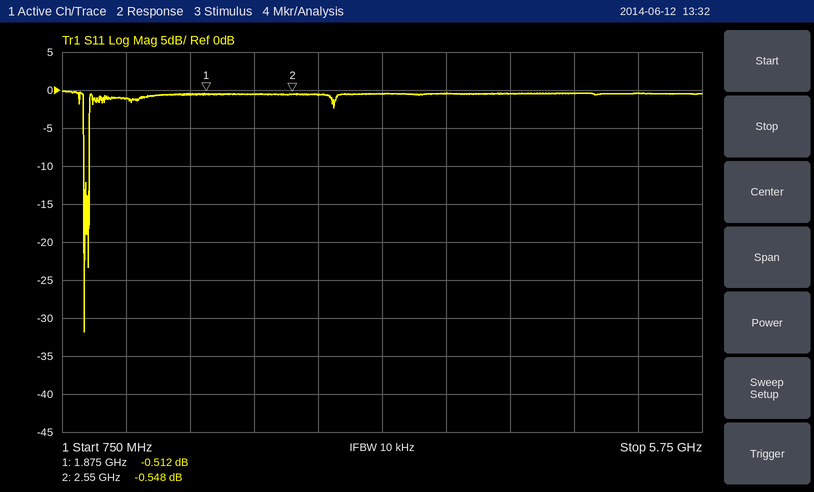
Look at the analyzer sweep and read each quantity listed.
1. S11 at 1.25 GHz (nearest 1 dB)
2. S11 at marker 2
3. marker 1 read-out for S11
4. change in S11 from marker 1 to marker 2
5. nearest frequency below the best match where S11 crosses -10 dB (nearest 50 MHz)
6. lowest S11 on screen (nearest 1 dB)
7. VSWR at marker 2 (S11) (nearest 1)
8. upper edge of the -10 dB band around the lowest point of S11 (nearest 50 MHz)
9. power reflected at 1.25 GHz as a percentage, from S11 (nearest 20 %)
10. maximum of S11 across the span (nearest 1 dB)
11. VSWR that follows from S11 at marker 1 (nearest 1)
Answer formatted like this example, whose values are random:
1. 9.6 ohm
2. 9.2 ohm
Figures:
1. -1 dB
2. -0.548 dB
3. -0.512 dB
4. -0.036 dB
5. 900 MHz
6. -32 dB
7. 32
8. 950 MHz
9. 80 %
10. 0 dB
11. 34
